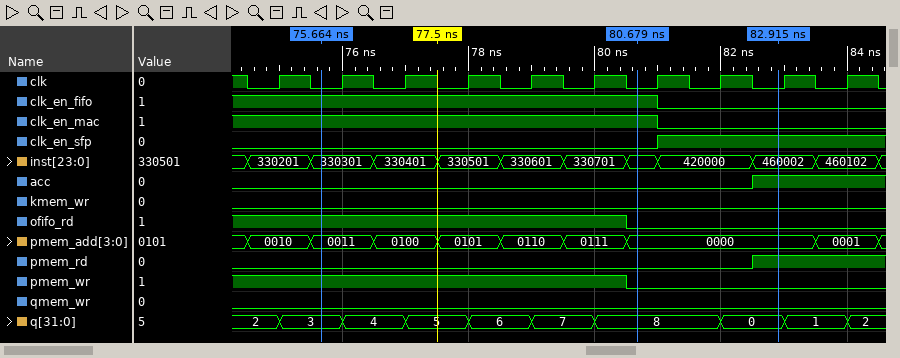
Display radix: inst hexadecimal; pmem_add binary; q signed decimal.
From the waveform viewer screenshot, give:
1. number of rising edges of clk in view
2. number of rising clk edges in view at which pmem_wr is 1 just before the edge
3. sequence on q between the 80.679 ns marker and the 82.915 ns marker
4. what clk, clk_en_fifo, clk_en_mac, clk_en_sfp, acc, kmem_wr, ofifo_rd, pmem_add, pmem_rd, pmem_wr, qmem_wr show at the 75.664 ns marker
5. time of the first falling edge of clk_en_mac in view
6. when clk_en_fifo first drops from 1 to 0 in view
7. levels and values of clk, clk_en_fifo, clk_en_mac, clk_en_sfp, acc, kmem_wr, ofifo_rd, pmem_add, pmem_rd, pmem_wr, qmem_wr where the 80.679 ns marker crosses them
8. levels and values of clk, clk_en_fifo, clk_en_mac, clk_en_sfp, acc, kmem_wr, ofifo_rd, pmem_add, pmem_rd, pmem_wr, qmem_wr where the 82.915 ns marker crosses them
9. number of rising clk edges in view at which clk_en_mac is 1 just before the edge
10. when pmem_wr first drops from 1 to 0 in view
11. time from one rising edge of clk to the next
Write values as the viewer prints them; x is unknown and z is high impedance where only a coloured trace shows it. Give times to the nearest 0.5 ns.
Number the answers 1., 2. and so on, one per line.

1. 10
2. 6
3. 8, 0
4. clk=0, clk_en_fifo=1, clk_en_mac=1, clk_en_sfp=0, acc=0, kmem_wr=0, ofifo_rd=1, pmem_add=0011, pmem_rd=0, pmem_wr=1, qmem_wr=0
5. 81 ns
6. 81 ns
7. clk=0, clk_en_fifo=1, clk_en_mac=1, clk_en_sfp=0, acc=0, kmem_wr=0, ofifo_rd=0, pmem_add=0000, pmem_rd=0, pmem_wr=0, qmem_wr=0
8. clk=0, clk_en_fifo=0, clk_en_mac=0, clk_en_sfp=1, acc=1, kmem_wr=0, ofifo_rd=0, pmem_add=0000, pmem_rd=1, pmem_wr=0, qmem_wr=0
9. 7
10. 80.5 ns
11. 1 ns
